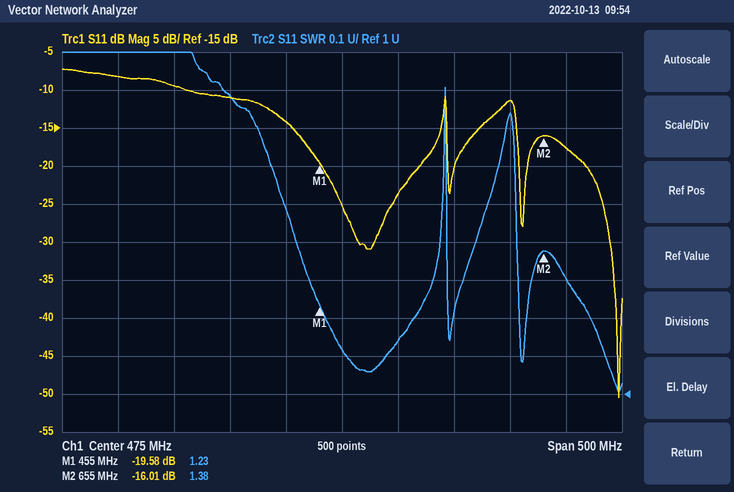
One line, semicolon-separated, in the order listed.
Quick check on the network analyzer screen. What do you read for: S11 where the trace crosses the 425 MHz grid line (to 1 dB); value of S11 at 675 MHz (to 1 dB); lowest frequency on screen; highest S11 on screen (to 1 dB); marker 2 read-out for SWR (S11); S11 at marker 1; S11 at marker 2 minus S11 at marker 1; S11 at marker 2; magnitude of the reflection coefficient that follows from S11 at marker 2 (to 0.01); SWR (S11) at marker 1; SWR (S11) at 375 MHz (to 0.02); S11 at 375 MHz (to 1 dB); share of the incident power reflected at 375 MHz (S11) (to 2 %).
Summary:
-14 dB; -18 dB; 225 MHz; -7 dB; 1.38; -19.58 dB; 3.57 dB; -16.01 dB; 0.16; 1.23; 1.78; -11 dB; 8 %
